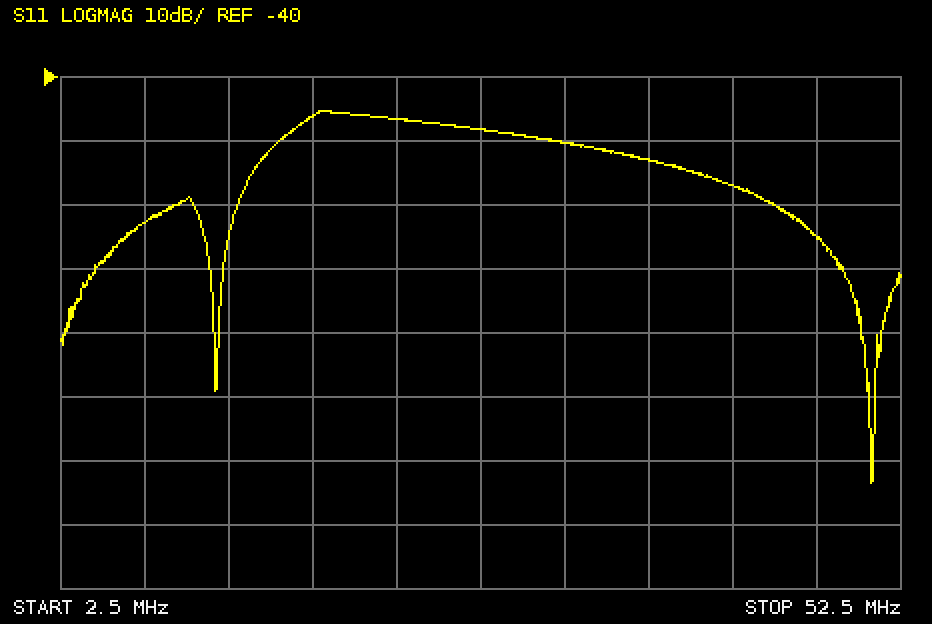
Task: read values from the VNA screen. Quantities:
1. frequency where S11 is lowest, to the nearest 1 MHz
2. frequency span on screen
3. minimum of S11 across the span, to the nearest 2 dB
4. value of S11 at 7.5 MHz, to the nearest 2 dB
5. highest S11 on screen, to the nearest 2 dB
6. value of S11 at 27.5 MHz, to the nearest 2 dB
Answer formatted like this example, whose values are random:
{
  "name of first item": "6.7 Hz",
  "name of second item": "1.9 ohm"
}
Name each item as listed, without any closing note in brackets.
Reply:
{
  "frequency where S11 is lowest, to the nearest 1 MHz": "51 MHz",
  "frequency span on screen": "50 MHz",
  "minimum of S11 across the span, to the nearest 2 dB": "-104 dB",
  "value of S11 at 7.5 MHz, to the nearest 2 dB": "-62 dB",
  "highest S11 on screen, to the nearest 2 dB": "-46 dB",
  "value of S11 at 27.5 MHz, to the nearest 2 dB": "-48 dB"
}
